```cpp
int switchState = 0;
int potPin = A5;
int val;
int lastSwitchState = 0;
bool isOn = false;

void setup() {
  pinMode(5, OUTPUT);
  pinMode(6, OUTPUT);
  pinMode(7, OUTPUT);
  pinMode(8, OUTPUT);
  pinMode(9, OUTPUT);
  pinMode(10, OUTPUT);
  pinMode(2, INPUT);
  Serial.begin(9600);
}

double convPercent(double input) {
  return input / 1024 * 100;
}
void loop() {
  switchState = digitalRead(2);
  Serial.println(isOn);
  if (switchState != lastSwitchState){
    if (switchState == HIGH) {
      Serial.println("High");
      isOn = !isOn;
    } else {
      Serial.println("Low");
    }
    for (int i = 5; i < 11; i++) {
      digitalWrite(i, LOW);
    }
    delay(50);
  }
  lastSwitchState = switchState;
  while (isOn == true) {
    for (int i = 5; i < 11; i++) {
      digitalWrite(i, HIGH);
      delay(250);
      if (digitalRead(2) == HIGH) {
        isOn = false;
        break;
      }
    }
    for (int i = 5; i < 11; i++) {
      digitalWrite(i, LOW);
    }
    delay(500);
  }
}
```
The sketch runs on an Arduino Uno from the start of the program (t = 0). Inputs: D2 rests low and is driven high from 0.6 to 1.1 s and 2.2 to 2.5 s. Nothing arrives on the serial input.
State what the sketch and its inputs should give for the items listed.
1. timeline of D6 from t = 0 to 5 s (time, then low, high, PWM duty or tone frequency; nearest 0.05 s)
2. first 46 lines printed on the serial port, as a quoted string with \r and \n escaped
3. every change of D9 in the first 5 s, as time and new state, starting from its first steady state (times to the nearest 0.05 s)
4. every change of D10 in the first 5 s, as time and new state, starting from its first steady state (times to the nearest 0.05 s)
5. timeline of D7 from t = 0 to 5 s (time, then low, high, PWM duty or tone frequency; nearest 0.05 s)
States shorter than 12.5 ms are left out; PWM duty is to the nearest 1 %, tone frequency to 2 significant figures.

0 s low; 2.5 s high; 3.75 s low; 4.5 s high
"0\r\n0\r\n0\r\n0\r\n0\r\n0\r\n0\r\n0\r\n0\r\n0\r\n0\r\n0\r\n0\r\n0\r\n0\r\n0\r\n0\r\n0\r\n0\r\n0\r\n0\r\n0\r\n0\r\n0\r\n0\r\n0\r\n0\r\n0\r\n0\r\n0\r\n0\r\n0\r\n0\r\n0\r\n0\r\n0\r\n0\r\n0\r\n0\r\n0\r\n0\r\n0\r\n0\r\n0\r\n0\r\n0\r\n"
0 s low; 3.25 s high; 3.75 s low
0 s low; 3.5 s high; 3.75 s low
0 s low; 2.75 s high; 3.75 s low; 4.75 s high
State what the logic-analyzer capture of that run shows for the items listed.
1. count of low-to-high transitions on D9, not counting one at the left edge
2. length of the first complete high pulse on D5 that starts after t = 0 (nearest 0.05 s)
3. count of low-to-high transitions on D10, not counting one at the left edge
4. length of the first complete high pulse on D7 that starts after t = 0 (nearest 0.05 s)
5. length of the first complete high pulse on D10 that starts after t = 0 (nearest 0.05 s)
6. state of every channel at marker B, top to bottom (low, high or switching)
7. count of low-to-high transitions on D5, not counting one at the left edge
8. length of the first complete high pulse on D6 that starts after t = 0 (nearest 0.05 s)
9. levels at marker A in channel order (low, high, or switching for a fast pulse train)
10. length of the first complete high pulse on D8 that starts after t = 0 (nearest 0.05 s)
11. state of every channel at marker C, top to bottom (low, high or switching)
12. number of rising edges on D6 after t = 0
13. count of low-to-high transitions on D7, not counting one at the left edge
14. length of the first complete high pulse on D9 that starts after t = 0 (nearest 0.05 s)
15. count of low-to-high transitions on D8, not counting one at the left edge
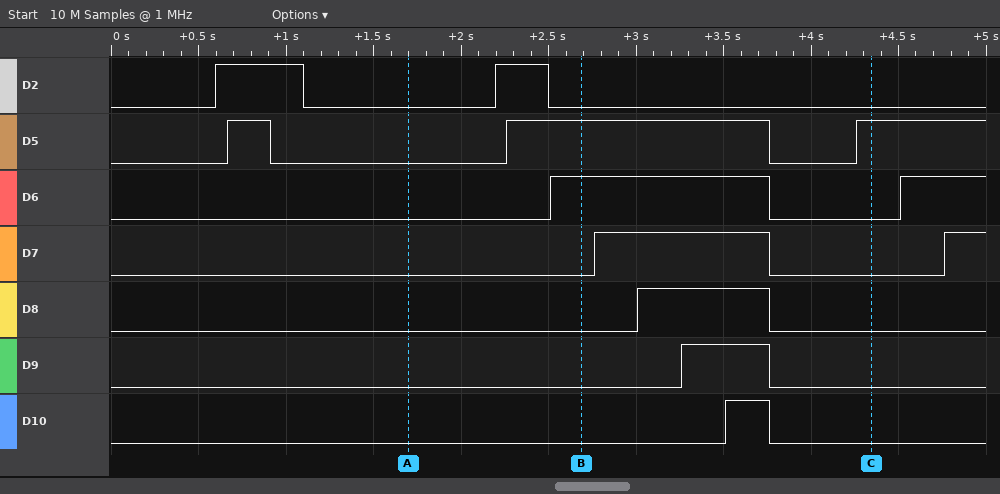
1
0.25 s
1
1.00 s
0.25 s
D2 low, D5 high, D6 high, D7 low, D8 low, D9 low, D10 low
3
1.25 s
D2 low, D5 low, D6 low, D7 low, D8 low, D9 low, D10 low
0.75 s
D2 low, D5 high, D6 low, D7 low, D8 low, D9 low, D10 low
2
2
0.50 s
1
